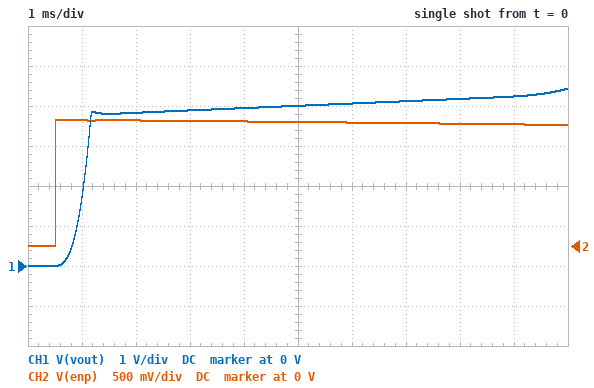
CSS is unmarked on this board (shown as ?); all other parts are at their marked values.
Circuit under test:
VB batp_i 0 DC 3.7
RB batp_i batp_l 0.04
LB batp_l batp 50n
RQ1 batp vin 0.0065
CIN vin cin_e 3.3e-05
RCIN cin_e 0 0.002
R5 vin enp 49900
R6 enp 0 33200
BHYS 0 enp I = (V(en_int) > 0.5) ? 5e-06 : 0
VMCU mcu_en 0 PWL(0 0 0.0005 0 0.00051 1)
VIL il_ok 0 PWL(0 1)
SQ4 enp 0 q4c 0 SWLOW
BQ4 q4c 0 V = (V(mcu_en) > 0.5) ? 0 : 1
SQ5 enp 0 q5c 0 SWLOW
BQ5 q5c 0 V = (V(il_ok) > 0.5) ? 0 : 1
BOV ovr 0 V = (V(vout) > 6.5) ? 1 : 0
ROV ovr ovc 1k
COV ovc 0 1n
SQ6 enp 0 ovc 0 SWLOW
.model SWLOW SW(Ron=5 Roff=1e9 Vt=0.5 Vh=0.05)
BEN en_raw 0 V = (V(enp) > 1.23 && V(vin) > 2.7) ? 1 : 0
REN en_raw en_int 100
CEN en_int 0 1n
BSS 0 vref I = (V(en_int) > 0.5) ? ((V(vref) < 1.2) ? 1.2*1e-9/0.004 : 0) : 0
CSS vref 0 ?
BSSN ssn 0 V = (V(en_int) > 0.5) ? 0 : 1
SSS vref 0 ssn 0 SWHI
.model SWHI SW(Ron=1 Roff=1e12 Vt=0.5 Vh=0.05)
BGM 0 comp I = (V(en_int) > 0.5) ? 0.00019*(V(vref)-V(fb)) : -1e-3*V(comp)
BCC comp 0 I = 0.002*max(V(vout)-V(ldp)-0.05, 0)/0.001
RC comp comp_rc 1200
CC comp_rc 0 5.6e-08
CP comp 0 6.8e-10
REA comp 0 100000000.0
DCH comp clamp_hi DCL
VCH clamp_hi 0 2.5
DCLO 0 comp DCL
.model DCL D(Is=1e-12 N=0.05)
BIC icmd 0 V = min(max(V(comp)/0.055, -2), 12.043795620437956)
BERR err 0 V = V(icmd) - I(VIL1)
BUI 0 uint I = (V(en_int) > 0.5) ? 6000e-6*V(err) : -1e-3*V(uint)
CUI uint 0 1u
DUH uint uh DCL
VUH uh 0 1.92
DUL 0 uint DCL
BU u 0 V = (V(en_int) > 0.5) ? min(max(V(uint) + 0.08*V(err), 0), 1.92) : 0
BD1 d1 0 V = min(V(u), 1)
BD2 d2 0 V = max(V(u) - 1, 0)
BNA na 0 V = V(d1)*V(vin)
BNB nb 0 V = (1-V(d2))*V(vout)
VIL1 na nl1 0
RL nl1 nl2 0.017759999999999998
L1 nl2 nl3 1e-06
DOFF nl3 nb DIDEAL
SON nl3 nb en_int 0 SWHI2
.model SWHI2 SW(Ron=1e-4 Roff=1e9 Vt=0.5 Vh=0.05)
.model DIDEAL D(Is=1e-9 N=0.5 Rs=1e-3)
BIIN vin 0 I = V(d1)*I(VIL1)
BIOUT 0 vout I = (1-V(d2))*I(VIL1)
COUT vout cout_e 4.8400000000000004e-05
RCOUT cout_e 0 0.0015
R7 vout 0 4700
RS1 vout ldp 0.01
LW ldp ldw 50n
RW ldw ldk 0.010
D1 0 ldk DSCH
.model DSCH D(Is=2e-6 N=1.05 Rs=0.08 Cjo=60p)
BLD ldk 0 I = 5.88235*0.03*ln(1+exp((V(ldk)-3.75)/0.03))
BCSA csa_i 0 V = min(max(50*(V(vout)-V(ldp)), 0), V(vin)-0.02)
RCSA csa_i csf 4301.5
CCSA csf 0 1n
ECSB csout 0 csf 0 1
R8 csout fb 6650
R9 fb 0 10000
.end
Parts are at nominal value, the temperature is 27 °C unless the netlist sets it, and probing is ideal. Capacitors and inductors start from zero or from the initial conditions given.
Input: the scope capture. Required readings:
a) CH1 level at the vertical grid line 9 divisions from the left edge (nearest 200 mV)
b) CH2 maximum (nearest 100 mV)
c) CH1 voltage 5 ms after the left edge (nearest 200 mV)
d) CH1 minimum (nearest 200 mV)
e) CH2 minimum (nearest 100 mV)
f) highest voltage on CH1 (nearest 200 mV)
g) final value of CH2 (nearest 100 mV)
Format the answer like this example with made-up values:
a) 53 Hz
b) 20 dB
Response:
a) 4.2 V
b) 1.6 V
c) 4.0 V
d) 0 V
e) 0 V
f) 4.4 V
g) 1.5 V
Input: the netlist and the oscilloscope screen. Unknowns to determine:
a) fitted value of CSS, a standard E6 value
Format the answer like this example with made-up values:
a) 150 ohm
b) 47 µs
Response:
a) 3.3 nF
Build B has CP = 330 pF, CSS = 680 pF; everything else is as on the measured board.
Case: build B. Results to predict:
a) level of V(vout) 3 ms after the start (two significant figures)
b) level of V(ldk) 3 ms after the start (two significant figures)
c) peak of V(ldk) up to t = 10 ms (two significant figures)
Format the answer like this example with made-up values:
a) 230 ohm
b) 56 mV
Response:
a) 6.1 V
b) 6.0 V
c) 6.5 V
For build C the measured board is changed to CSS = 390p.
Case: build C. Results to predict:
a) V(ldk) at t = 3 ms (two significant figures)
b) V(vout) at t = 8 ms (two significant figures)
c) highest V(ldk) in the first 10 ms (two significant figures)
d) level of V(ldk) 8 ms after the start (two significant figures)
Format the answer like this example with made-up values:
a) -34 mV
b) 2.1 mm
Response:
a) 4.1 V
b) 4.5 V
c) 6.5 V
d) 4.4 V
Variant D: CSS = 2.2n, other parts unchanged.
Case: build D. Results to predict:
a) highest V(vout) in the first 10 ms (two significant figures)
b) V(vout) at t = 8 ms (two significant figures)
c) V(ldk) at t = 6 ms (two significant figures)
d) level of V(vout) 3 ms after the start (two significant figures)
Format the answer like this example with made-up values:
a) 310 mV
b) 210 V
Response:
a) 6.5 V
b) 6.1 V
c) 4.2 V
d) 4.0 V
